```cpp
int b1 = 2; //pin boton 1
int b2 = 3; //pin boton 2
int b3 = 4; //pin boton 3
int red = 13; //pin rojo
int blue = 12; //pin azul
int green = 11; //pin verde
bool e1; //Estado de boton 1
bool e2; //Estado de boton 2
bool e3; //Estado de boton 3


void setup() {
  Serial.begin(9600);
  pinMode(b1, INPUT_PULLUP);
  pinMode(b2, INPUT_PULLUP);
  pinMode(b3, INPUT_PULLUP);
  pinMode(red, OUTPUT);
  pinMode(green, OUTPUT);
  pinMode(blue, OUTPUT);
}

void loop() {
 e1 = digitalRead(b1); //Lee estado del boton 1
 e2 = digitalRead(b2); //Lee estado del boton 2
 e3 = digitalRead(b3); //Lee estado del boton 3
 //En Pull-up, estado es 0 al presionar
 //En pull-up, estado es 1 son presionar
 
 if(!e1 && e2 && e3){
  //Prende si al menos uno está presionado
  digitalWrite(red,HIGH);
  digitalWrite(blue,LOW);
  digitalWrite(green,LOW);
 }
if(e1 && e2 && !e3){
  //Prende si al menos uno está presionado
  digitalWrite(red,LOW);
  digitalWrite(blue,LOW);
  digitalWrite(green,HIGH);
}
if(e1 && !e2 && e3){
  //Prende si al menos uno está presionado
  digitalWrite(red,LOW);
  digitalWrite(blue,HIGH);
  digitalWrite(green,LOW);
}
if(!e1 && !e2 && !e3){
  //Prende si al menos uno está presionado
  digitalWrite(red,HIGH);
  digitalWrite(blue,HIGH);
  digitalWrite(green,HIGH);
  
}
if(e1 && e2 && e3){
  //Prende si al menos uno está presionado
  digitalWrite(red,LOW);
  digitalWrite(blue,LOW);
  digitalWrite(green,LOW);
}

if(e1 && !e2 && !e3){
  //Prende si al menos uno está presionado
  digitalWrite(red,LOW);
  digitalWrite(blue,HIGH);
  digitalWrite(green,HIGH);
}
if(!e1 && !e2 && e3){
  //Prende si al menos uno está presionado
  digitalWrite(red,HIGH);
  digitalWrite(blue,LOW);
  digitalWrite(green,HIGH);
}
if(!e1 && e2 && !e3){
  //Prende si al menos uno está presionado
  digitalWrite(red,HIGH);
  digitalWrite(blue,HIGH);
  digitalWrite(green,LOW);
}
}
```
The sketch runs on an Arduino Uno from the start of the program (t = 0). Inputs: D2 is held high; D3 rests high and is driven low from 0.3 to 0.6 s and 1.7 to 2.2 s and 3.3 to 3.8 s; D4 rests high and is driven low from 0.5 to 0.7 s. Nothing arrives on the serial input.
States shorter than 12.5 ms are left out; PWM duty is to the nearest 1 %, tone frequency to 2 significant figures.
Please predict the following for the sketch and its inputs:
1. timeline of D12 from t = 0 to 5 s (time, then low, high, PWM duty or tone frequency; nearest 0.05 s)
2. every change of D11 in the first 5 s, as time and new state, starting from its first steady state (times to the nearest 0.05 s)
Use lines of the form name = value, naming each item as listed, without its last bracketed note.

timeline of D12 from t = 0 to 5 s = 0 s low; 0.3 s high; 0.6 s low; 1.7 s high; 2.2 s low; 3.3 s high; 3.8 s low
every change of D11 in the first 5 s, as time and new state, starting from its first steady state = 0 s low; 0.5 s high; 0.7 s low
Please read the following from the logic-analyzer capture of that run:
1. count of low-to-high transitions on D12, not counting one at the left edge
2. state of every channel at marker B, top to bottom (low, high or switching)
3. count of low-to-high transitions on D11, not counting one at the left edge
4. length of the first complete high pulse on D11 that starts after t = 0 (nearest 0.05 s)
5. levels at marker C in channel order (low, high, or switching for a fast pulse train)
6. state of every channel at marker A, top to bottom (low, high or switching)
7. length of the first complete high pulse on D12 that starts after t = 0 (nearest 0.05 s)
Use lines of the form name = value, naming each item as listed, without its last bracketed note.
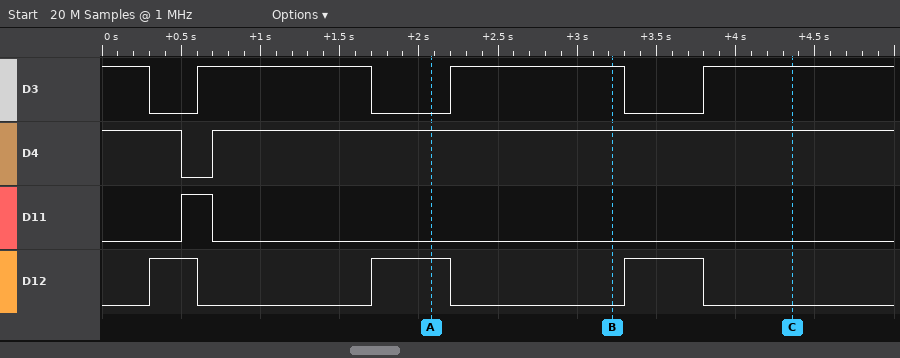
count of low-to-high transitions on D12, not counting one at the left edge = 3
state of every channel at marker B, top to bottom = D3 high, D4 high, D11 low, D12 low
count of low-to-high transitions on D11, not counting one at the left edge = 1
length of the first complete high pulse on D11 that starts after t = 0 = 0.20 s
levels at marker C in channel order = D3 high, D4 high, D11 low, D12 low
state of every channel at marker A, top to bottom = D3 low, D4 high, D11 low, D12 high
length of the first complete high pulse on D12 that starts after t = 0 = 0.30 s
